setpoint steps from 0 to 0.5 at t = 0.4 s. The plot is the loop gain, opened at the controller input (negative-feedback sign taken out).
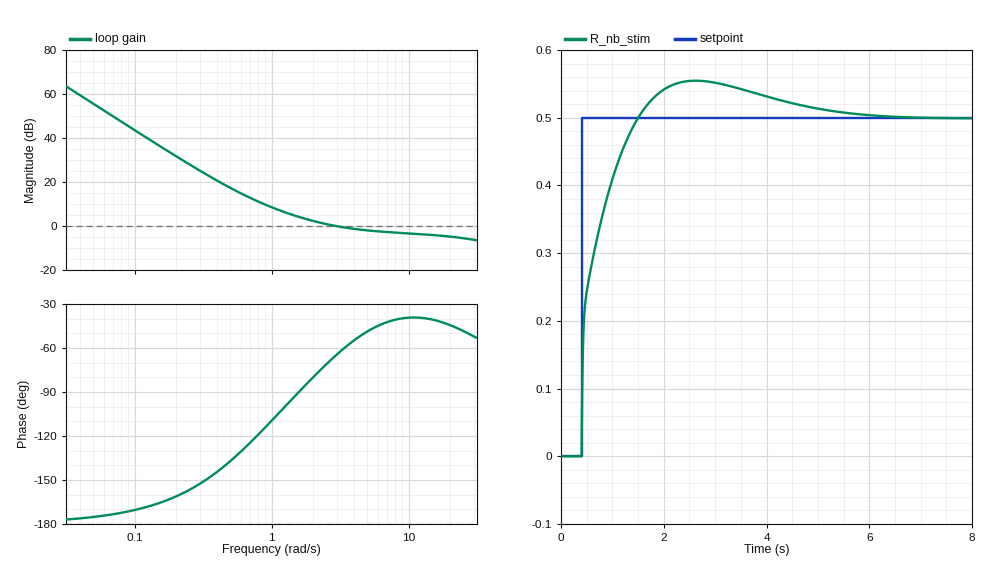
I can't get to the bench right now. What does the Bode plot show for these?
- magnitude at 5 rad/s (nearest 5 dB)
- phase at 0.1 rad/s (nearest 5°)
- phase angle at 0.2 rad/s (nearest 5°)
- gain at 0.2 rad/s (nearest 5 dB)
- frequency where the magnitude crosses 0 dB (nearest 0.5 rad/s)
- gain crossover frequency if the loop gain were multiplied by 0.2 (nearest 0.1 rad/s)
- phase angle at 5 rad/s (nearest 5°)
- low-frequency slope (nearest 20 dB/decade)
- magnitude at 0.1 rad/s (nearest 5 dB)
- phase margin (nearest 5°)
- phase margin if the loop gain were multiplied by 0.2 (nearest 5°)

0 dB
-170°
-160°
30 dB
3.0 rad/s
0.6 rad/s
-50°
-40 dB/decade
45 dB
115°
50°
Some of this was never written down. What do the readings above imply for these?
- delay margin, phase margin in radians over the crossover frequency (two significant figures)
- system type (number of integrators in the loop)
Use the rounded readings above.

0.67 s
2
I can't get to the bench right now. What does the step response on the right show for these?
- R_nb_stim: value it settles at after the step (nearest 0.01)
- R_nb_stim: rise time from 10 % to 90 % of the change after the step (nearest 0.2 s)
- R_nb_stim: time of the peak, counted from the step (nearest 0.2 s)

0.50
0.8 s
2.2 s
